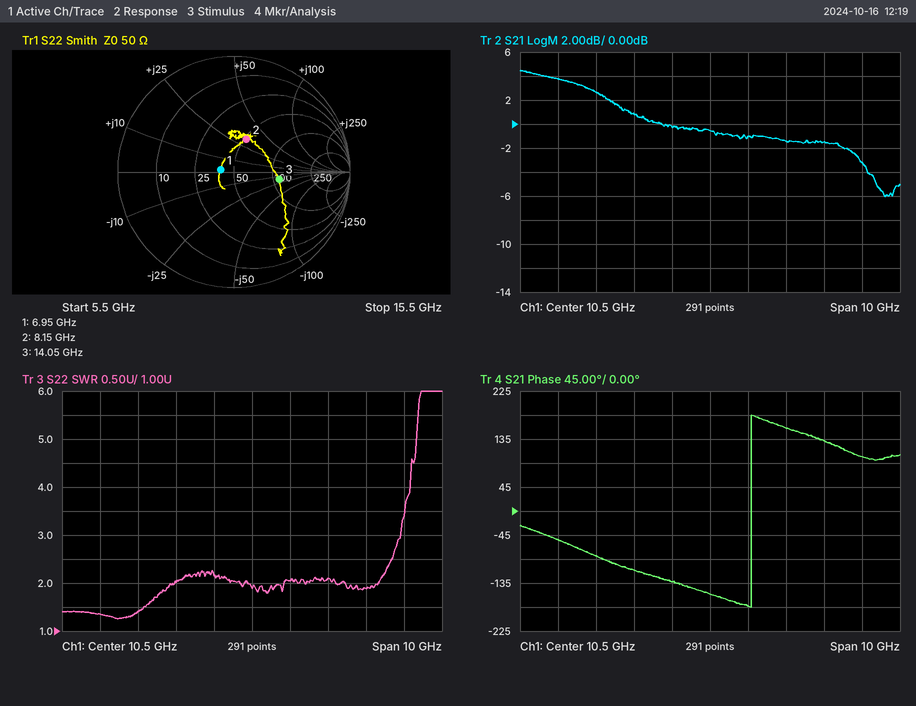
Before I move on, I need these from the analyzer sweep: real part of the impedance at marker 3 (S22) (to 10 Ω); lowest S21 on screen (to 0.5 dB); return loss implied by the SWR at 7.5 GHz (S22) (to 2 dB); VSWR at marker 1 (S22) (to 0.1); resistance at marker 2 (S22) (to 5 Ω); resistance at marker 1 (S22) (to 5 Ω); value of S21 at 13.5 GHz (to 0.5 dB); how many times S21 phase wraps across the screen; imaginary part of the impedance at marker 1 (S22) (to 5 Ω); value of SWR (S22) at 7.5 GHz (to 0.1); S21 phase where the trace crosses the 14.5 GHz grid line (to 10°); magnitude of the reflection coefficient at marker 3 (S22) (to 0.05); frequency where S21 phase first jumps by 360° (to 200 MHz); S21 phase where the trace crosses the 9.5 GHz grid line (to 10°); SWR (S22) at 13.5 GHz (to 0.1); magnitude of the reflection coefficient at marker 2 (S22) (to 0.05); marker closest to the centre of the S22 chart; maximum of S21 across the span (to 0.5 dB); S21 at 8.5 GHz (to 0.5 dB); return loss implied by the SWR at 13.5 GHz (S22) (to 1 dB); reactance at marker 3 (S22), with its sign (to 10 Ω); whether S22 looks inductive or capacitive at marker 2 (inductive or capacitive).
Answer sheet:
110 Ω
-6.0 dB
16 dB
1.3
50 Ω
40 Ω
-1.5 dB
1
0 Ω
1.4
100°
0.40
11.6 GHz
-130°
1.9
0.30
marker 1
4.5 dB
1.0 dB
10 dB
-20 Ω
inductive
